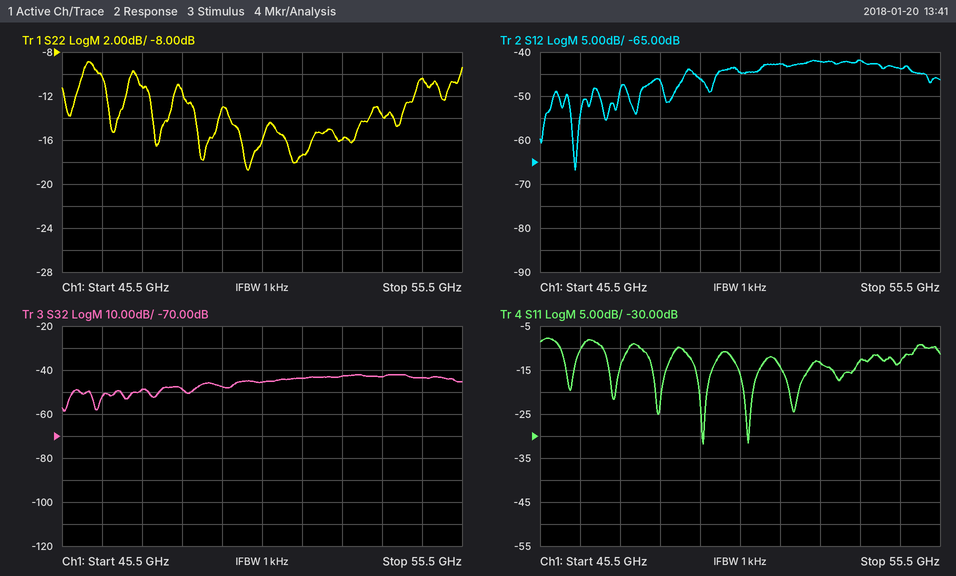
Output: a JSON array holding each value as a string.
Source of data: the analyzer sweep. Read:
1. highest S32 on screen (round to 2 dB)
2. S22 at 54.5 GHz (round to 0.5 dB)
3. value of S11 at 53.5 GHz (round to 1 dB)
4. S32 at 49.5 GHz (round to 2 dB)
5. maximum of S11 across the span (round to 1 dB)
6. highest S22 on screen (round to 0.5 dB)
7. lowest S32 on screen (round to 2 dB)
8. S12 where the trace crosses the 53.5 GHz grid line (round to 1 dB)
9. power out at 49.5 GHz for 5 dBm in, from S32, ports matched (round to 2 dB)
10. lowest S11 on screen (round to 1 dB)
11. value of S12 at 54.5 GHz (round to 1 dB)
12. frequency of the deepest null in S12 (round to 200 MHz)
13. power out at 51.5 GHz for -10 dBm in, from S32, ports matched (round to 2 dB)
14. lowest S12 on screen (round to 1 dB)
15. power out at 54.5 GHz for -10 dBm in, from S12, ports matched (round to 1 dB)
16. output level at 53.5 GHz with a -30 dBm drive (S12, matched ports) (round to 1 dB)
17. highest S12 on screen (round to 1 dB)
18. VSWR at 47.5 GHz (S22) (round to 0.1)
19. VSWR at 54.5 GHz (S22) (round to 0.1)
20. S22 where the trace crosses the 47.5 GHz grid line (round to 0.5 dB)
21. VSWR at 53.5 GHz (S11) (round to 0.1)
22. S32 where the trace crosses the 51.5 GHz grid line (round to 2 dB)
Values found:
["-42 dB", "-10.5 dB", "-13 dB", "-48 dB", "-8 dB", "-9.0 dB", "-58 dB", "-42 dB", "-42 dBm", "-32 dB", "-44 dB", "46.4 GHz", "-54 dBm", "-67 dB", "-54 dBm", "-72 dBm", "-42 dB", "1.8", "1.9", "-11.0 dB", "1.6", "-44 dB"]
